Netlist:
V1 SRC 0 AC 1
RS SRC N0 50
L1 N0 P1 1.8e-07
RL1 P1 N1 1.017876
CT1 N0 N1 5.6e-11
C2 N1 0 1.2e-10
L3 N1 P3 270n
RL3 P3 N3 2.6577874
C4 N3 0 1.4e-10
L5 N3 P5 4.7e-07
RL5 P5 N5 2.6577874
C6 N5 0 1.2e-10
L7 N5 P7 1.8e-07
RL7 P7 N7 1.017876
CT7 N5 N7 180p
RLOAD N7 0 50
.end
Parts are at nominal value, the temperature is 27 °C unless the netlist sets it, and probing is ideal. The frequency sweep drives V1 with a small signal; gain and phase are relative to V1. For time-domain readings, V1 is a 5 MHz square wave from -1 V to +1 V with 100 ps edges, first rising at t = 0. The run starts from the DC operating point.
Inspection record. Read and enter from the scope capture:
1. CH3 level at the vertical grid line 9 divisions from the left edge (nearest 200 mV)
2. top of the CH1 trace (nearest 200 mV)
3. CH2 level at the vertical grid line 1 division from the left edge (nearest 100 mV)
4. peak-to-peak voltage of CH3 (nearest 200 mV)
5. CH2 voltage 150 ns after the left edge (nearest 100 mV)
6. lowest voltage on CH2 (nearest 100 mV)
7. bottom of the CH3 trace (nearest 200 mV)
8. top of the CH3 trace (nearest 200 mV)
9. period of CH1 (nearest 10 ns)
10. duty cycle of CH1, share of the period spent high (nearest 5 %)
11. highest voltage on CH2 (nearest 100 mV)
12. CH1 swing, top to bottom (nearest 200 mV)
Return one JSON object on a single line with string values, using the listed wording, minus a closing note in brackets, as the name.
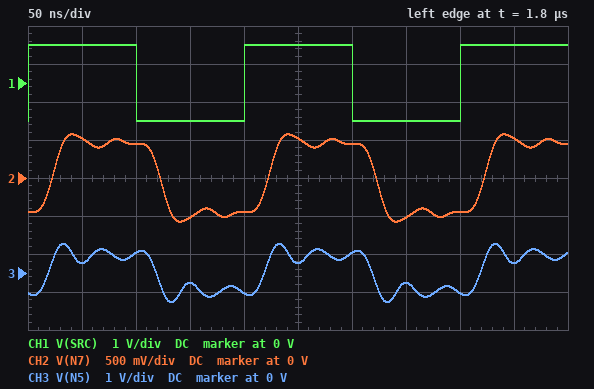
{"CH3 level at the vertical grid line 9 divisions from the left edge": "200 mV", "top of the CH1 trace": "1.0 V", "CH2 level at the vertical grid line 1 division from the left edge": "500 mV", "peak-to-peak voltage of CH3": "1.6 V", "CH2 voltage 150 ns after the left edge": "-500 mV", "lowest voltage on CH2": "-600 mV", "bottom of the CH3 trace": "-800 mV", "top of the CH3 trace": "800 mV", "period of CH1": "200 ns", "duty cycle of CH1, share of the period spent high": "50 %", "highest voltage on CH2": "600 mV", "CH1 swing, top to bottom": "2.0 V"}
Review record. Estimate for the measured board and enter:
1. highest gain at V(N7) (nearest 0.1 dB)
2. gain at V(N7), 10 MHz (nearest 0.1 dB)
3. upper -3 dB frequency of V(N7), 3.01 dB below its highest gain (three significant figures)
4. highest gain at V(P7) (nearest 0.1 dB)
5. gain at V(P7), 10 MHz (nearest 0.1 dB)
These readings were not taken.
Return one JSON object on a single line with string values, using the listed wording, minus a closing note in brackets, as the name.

{"highest gain at V(N7)": "-6.6 dB", "gain at V(N7), 10 MHz": "-6.7 dB", "upper -3 dB frequency of V(N7), 3.01 dB below its highest gain": "24.6 MHz", "highest gain at V(P7)": "-6.5 dB", "gain at V(P7), 10 MHz": "-6.5 dB"}
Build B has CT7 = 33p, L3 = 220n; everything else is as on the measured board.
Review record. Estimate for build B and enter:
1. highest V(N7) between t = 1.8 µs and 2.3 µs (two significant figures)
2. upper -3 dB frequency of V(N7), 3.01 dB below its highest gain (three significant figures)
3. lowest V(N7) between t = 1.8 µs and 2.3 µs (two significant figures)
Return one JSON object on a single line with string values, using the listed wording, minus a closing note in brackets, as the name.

{"highest V(N7) between t = 1.8 µs and 2.3 µs": "600 mV", "upper -3 dB frequency of V(N7), 3.01 dB below its highest gain": "32.0 MHz", "lowest V(N7) between t = 1.8 µs and 2.3 µs": "-600 mV"}
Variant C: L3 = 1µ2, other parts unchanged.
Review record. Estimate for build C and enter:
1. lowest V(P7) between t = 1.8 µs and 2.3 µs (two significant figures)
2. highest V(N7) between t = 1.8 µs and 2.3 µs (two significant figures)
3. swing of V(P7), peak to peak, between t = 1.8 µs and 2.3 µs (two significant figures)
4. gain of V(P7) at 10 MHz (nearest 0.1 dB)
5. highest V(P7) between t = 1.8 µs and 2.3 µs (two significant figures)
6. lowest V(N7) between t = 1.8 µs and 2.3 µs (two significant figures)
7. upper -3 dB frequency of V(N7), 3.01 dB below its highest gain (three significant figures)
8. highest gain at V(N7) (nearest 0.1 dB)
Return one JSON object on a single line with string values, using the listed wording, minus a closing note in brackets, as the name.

{"lowest V(P7) between t = 1.8 µs and 2.3 µs": "-540 mV", "highest V(N7) between t = 1.8 µs and 2.3 µs": "520 mV", "swing of V(P7), peak to peak, between t = 1.8 µs and 2.3 µs": "1.1 V", "gain of V(P7) at 10 MHz": "-7.3 dB", "highest V(P7) between t = 1.8 µs and 2.3 µs": "540 mV", "lowest V(N7) between t = 1.8 µs and 2.3 µs": "-520 mV", "upper -3 dB frequency of V(N7), 3.01 dB below its highest gain": "19.7 MHz", "highest gain at V(N7)": "-6.6 dB"}
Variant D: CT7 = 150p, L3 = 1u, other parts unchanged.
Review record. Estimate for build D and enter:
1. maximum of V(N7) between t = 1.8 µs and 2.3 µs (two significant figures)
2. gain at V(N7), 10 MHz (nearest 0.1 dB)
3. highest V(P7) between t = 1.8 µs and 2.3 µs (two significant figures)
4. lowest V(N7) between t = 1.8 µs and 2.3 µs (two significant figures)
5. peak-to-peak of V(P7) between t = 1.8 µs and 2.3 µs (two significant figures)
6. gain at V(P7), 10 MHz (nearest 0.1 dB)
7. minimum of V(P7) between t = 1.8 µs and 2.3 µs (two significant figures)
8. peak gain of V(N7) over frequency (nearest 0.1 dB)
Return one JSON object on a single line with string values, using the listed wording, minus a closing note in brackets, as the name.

{"maximum of V(N7) between t = 1.8 µs and 2.3 µs": "550 mV", "gain at V(N7), 10 MHz": "-7.2 dB", "highest V(P7) between t = 1.8 µs and 2.3 µs": "570 mV", "lowest V(N7) between t = 1.8 µs and 2.3 µs": "-550 mV", "peak-to-peak of V(P7) between t = 1.8 µs and 2.3 µs": "1.1 V", "gain at V(P7), 10 MHz": "-7.0 dB", "minimum of V(P7) between t = 1.8 µs and 2.3 µs": "-570 mV", "peak gain of V(N7) over frequency": "-6.6 dB"}
